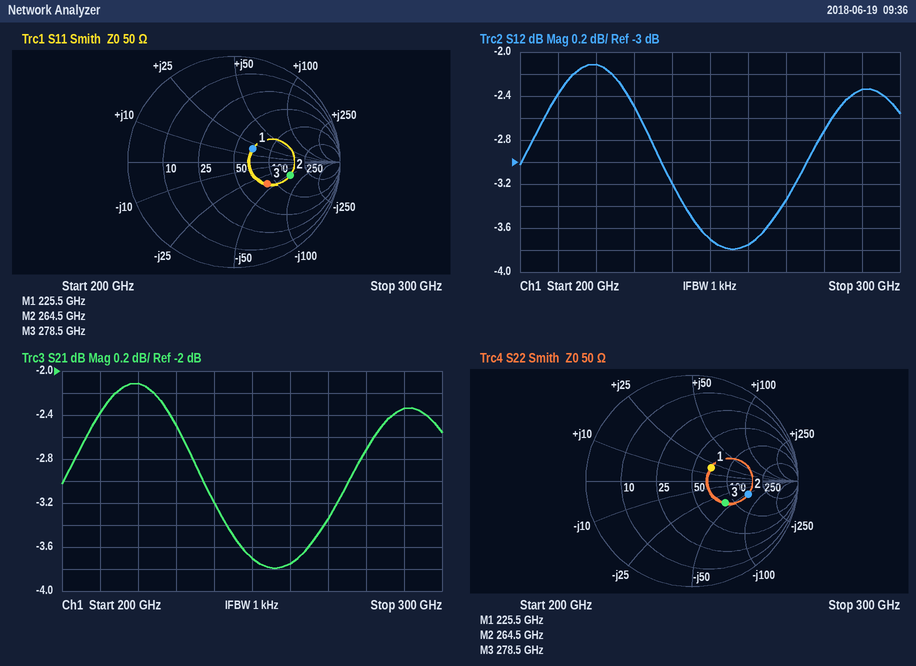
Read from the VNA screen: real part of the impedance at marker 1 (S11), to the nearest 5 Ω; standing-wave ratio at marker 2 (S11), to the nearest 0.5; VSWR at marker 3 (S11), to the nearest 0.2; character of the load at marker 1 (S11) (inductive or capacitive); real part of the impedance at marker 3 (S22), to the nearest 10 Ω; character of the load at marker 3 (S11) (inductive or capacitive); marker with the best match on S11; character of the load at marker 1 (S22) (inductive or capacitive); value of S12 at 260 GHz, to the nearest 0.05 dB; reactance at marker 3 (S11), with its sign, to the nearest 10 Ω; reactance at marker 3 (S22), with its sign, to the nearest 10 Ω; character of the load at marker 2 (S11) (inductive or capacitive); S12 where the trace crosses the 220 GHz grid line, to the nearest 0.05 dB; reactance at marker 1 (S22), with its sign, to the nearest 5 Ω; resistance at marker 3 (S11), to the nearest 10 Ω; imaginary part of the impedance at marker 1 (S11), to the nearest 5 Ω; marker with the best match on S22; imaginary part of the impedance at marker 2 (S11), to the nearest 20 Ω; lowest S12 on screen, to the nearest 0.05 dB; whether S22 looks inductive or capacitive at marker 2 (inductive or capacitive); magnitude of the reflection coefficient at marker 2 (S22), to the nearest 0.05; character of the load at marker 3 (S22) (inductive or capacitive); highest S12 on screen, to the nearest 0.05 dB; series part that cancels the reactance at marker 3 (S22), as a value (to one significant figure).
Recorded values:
70 Ω
3.5
2.2
inductive
80 Ω
capacitive
marker 1
inductive
-3.75 dB
-40 Ω
-40 Ω
capacitive
-2.10 dB
+20 Ω
80 Ω
+20 Ω
marker 1
-60 Ω
-3.80 dB
capacitive
0.55
capacitive
-2.10 dB
20 pH
